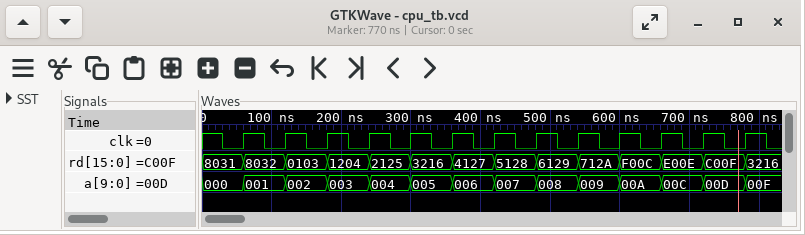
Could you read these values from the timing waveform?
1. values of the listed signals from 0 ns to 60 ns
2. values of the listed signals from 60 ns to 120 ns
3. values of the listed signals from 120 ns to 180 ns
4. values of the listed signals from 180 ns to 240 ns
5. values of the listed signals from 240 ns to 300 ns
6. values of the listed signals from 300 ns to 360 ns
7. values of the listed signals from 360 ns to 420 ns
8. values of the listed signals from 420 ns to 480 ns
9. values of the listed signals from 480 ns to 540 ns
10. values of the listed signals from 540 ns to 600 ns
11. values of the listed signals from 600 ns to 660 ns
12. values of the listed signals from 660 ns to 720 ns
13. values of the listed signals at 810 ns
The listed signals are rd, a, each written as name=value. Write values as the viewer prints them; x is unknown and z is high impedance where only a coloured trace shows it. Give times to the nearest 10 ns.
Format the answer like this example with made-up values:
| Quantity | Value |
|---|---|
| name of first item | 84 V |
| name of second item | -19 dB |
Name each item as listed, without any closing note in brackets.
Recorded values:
| Quantity | Value |
|---|---|
| values of the listed signals from 0 ns to 60 ns | rd=8031, a=000 |
| values of the listed signals from 60 ns to 120 ns | rd=8032, a=001 |
| values of the listed signals from 120 ns to 180 ns | rd=0103, a=002 |
| values of the listed signals from 180 ns to 240 ns | rd=1204, a=003 |
| values of the listed signals from 240 ns to 300 ns | rd=2125, a=004 |
| values of the listed signals from 300 ns to 360 ns | rd=3216, a=005 |
| values of the listed signals from 360 ns to 420 ns | rd=4127, a=006 |
| values of the listed signals from 420 ns to 480 ns | rd=5128, a=007 |
| values of the listed signals from 480 ns to 540 ns | rd=6129, a=008 |
| values of the listed signals from 540 ns to 600 ns | rd=712A, a=009 |
| values of the listed signals from 600 ns to 660 ns | rd=F00C, a=00A |
| values of the listed signals from 660 ns to 720 ns | rd=E00E, a=00C |
| values of the listed signals at 810 ns | rd=3216, a=00F |
